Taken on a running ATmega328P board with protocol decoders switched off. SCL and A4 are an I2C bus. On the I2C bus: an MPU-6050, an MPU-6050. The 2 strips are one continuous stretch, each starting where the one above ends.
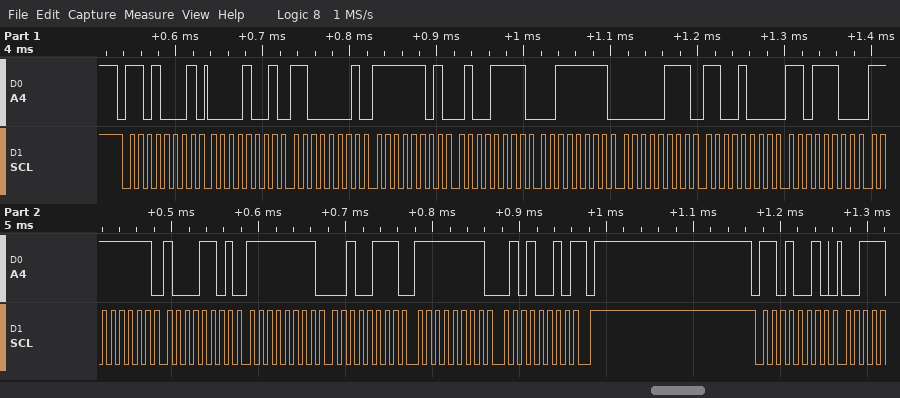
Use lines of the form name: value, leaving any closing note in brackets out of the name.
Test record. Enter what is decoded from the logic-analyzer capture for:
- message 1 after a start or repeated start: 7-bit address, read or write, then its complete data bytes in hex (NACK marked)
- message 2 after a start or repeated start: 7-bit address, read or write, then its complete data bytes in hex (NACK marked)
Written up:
message 1 after a start or repeated start: 7-bit address, read or write, then its complete data bytes in hex: 0x68 read: 09 C1 FD 4F 3F 07 C8 DC FF 8D FF 27 FF 52 NACK
message 2 after a start or repeated start: 7-bit address, read or write, then its complete data bytes in hex: 0x69 write
